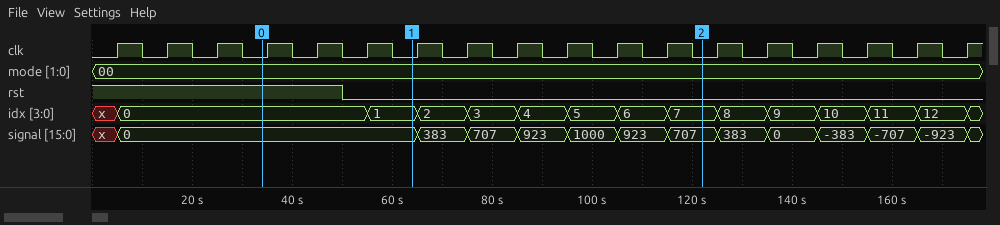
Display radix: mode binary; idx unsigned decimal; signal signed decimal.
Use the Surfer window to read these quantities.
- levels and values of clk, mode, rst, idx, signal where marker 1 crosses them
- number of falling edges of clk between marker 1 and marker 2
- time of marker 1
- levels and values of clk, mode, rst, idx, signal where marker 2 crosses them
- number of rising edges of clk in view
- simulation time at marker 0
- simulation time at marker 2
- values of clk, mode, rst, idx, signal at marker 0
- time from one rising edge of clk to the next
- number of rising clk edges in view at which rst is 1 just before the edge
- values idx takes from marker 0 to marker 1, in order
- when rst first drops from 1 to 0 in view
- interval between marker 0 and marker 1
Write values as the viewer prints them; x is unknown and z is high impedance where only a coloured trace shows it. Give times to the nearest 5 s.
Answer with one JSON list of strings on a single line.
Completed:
["clk=0, mode=00, rst=0, idx=1, signal=0", "6", "65 s", "clk=0, mode=00, rst=0, idx=7, signal=707", "18", "35 s", "120 s", "clk=0, mode=00, rst=1, idx=0, signal=0", "10 s", "5", "0, 1", "50 s", "30 s"]
